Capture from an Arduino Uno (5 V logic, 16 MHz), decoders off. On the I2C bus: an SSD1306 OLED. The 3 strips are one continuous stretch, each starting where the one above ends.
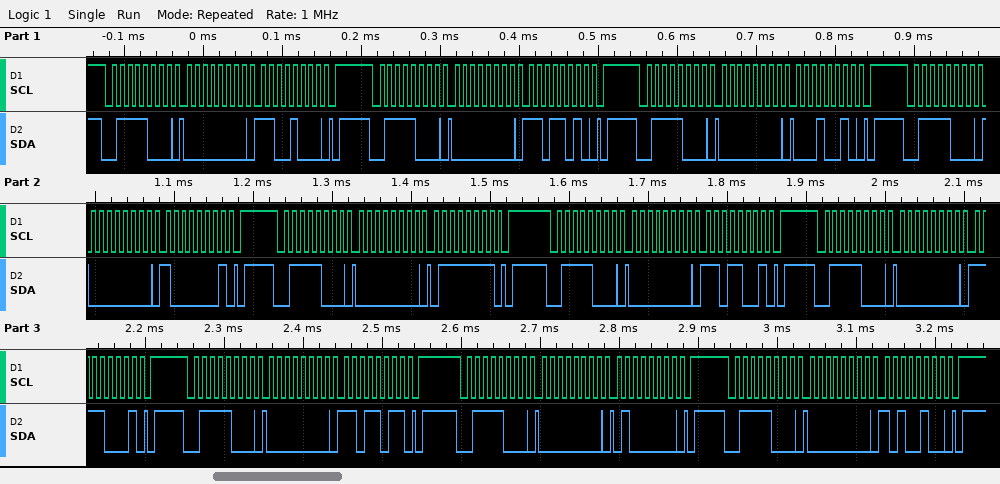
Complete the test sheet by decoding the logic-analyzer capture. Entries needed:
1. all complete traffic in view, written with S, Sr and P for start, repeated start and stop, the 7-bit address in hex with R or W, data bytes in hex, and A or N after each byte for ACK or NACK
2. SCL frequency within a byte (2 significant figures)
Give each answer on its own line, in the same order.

S 3CW A 00 A C8 A P S 3CW A 00 A DA A P S 3CW A 00 A 12 A P S 3CW A 00 A 81 A P S 3CW A 00 A 7F A P S 3CW A 00 A D9 A P S 3CW A 00 A F1 A P S 3CW A 00 A DB A P S 3CW A 00 A 40 A P S 3CW A 00 A A4 A P
100 kHz
